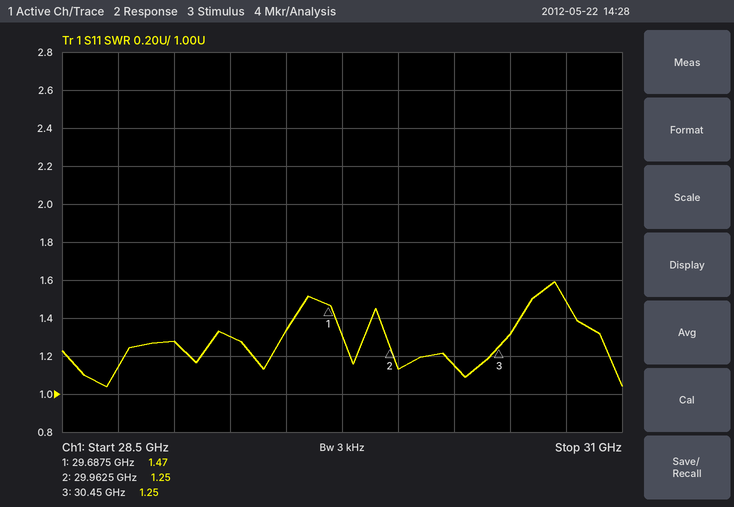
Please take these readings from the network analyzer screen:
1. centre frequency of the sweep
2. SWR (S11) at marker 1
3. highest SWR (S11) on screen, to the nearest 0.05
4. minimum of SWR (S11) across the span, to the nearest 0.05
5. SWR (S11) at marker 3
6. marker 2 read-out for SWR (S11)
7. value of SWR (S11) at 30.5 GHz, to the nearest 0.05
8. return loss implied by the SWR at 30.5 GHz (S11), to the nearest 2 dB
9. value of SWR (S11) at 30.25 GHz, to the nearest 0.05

29.75 GHz
1.47
1.60
1.05
1.25
1.25
1.30
18 dB
1.15
